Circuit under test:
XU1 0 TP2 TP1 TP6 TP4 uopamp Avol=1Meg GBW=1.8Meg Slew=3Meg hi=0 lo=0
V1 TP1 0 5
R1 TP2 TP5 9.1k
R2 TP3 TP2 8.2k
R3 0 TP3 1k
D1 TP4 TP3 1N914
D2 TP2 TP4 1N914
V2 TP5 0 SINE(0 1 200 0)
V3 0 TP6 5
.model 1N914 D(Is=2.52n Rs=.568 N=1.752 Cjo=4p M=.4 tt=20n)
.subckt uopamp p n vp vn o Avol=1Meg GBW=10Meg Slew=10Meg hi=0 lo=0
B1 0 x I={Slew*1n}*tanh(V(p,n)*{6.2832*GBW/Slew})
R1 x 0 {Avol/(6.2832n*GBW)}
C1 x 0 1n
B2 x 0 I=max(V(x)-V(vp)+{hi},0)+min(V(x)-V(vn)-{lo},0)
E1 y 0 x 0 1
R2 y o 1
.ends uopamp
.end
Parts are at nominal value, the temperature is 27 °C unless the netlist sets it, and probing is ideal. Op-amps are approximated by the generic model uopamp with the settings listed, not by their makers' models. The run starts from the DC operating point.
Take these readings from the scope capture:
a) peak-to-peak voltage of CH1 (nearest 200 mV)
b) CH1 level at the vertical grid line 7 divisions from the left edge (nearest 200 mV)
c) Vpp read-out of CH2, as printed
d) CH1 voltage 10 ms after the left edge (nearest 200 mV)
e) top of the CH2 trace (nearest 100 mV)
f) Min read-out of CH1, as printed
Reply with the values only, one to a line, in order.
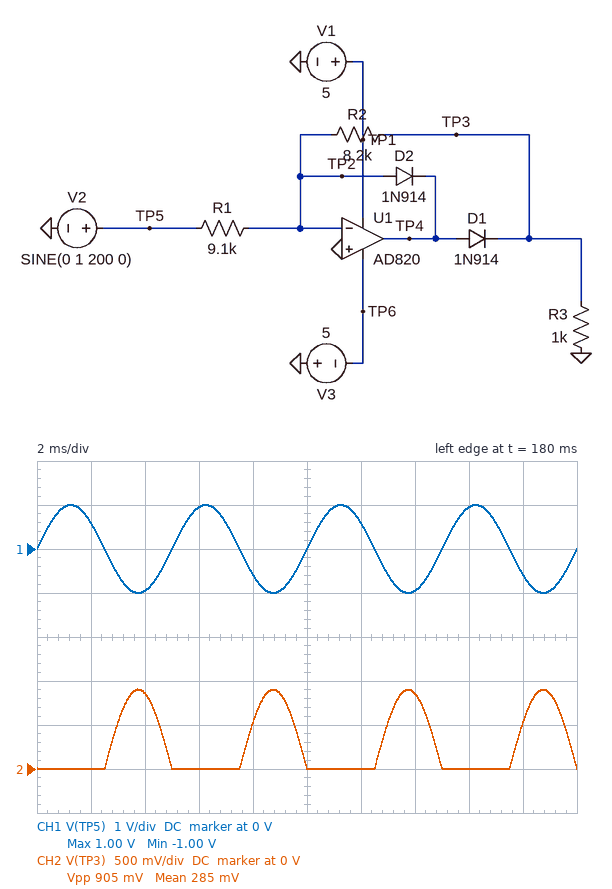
2.0 V
-1.0 V
905 mV
0 V
900 mV
-1.00 V
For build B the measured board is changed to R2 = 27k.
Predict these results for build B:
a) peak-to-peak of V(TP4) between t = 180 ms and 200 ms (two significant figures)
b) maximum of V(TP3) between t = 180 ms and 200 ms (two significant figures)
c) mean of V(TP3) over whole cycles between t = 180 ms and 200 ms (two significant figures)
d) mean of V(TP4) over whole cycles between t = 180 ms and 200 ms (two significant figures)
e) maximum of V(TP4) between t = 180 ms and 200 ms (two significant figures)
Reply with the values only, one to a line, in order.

4.1 V
3.0 V
940 mV
1.0 V
3.6 V
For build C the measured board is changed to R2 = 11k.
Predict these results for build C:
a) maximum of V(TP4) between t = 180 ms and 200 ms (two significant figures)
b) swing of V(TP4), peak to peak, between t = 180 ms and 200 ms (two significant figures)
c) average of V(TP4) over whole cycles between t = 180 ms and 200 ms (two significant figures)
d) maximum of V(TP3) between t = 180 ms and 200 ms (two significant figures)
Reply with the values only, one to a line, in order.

1.8 V
2.3 V
440 mV
1.2 V
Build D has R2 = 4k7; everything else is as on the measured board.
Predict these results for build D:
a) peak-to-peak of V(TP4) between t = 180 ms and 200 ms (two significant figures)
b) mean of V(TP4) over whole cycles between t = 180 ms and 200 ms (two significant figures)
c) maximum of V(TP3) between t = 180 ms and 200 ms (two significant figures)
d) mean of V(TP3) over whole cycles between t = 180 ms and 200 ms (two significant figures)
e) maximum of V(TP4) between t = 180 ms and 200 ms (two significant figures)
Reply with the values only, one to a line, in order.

1.6 V
200 mV
520 mV
160 mV
1.1 V
